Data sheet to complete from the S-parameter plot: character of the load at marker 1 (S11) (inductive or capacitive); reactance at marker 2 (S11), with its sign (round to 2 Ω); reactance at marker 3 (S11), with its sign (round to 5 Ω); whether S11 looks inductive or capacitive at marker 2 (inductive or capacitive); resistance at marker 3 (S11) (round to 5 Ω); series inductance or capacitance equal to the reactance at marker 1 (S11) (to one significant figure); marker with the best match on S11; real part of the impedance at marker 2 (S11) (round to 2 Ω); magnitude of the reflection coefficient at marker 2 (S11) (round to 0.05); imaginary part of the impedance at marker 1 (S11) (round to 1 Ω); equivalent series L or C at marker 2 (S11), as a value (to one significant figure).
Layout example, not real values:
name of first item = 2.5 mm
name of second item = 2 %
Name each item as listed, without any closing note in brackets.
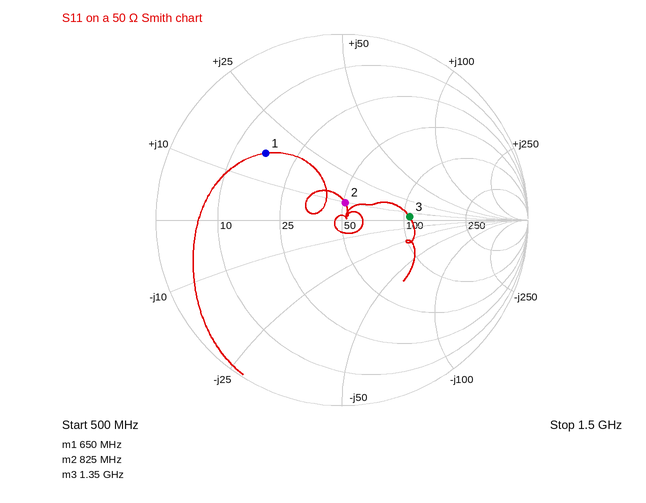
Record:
character of the load at marker 1 (S11) = inductive
reactance at marker 2 (S11), with its sign = +10 Ω
reactance at marker 3 (S11), with its sign = +5 Ω
whether S11 looks inductive or capacitive at marker 2 = inductive
resistance at marker 3 (S11) = 105 Ω
series inductance or capacitance equal to the reactance at marker 1 (S11) = 4 nH
marker with the best match on S11 = marker 2
real part of the impedance at marker 2 (S11) = 50 Ω
magnitude of the reflection coefficient at marker 2 (S11) = 0.10
imaginary part of the impedance at marker 1 (S11) = +17 Ω
equivalent series L or C at marker 2 (S11), as a value = 2 nH
